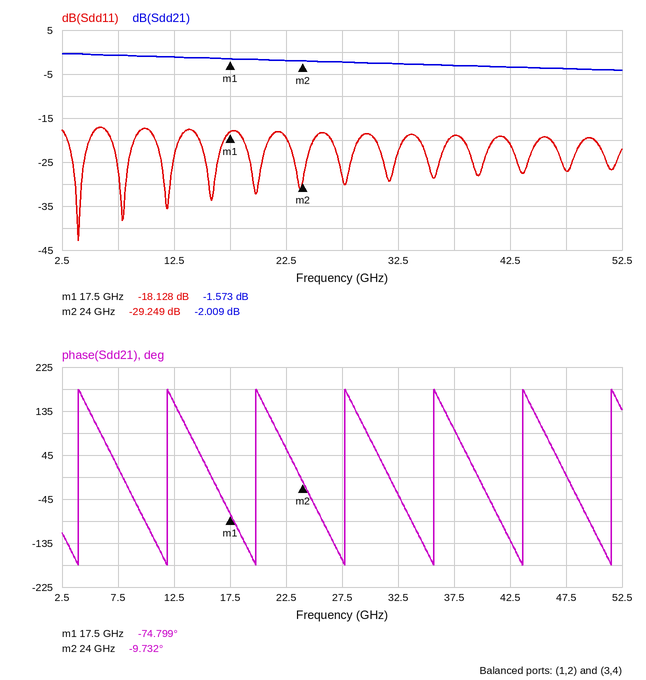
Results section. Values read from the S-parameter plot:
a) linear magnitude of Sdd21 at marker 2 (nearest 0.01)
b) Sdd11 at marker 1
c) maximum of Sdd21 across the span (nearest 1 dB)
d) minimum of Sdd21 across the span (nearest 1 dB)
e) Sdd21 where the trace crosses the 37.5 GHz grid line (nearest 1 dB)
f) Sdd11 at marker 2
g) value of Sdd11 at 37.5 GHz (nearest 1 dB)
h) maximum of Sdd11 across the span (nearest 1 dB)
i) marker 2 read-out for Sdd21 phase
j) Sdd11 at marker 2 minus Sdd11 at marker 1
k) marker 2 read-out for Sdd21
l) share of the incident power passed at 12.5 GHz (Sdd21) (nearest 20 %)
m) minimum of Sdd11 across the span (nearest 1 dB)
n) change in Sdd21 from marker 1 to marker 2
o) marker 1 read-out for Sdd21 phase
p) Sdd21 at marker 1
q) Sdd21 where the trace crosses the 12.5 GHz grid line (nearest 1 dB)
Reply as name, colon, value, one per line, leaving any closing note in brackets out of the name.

linear magnitude of Sdd21 at marker 2: 0.79
Sdd11 at marker 1: -18.128 dB
maximum of Sdd21 across the span: 0 dB
minimum of Sdd21 across the span: -4 dB
Sdd21 where the trace crosses the 37.5 GHz grid line: -3 dB
Sdd11 at marker 2: -29.249 dB
value of Sdd11 at 37.5 GHz: -19 dB
maximum of Sdd11 across the span: -17 dB
marker 2 read-out for Sdd21 phase: -9.732°
Sdd11 at marker 2 minus Sdd11 at marker 1: -11.121 dB
marker 2 read-out for Sdd21: -2.009 dB
share of the incident power passed at 12.5 GHz (Sdd21): 80 %
minimum of Sdd11 across the span: -43 dB
change in Sdd21 from marker 1 to marker 2: -0.436 dB
marker 1 read-out for Sdd21 phase: -74.799°
Sdd21 at marker 1: -1.573 dB
Sdd21 where the trace crosses the 12.5 GHz grid line: -1 dB
